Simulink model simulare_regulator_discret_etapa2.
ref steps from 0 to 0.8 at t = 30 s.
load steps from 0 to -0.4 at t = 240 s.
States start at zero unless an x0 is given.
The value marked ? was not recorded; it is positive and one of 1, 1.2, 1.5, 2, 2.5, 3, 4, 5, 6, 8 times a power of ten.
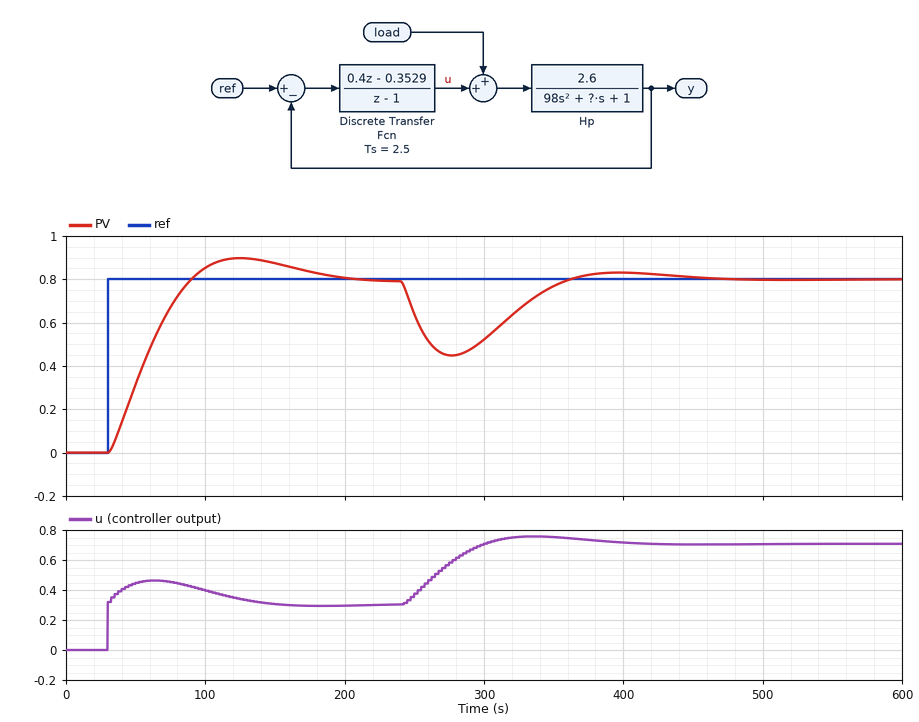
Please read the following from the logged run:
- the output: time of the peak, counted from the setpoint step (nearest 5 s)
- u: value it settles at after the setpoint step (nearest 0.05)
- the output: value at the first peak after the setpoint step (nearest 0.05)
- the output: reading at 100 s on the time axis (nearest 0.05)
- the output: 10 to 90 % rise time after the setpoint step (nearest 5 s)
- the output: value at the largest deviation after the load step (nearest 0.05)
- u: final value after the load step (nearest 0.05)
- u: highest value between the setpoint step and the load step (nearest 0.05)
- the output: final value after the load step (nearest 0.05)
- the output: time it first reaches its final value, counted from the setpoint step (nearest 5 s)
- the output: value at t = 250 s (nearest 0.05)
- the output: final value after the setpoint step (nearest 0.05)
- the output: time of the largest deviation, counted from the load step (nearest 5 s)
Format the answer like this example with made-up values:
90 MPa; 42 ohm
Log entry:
95 s; 0.30; 0.90; 0.85; 45 s; 0.45; 0.70; 0.45; 0.80; 60 s; 0.65; 0.80; 35 s
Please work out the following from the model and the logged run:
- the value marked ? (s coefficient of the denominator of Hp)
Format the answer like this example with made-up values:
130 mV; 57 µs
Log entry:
50
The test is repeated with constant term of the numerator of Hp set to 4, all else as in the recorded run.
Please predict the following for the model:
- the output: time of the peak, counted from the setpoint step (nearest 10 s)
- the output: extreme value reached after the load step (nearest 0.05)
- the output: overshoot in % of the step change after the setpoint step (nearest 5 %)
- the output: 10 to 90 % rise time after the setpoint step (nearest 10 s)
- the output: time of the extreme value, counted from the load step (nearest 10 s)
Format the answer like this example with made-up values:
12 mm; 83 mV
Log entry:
70 s; 0.35; 15 %; 30 s; 30 s
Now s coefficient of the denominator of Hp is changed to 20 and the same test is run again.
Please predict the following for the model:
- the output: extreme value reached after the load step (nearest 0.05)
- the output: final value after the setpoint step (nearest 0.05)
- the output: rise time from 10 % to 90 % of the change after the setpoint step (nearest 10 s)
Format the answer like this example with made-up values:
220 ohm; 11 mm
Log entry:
0.30; 0.80; 30 s
